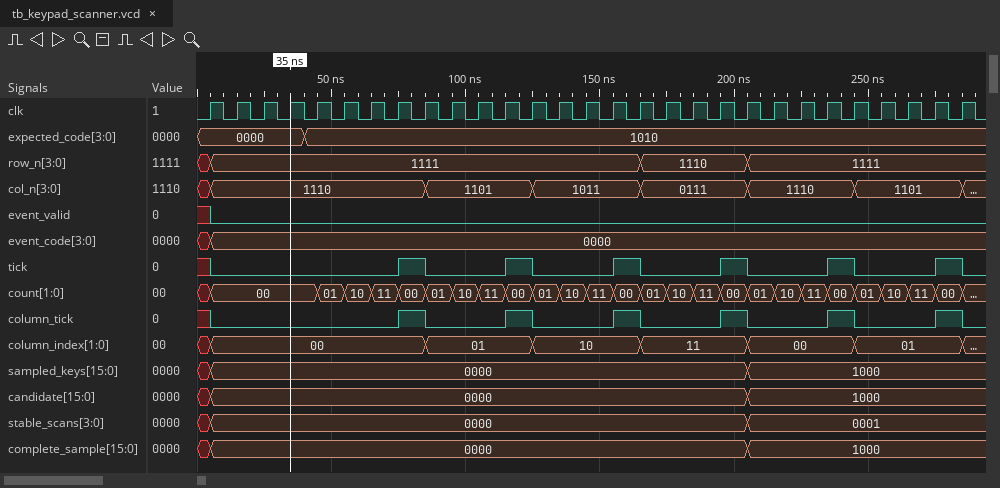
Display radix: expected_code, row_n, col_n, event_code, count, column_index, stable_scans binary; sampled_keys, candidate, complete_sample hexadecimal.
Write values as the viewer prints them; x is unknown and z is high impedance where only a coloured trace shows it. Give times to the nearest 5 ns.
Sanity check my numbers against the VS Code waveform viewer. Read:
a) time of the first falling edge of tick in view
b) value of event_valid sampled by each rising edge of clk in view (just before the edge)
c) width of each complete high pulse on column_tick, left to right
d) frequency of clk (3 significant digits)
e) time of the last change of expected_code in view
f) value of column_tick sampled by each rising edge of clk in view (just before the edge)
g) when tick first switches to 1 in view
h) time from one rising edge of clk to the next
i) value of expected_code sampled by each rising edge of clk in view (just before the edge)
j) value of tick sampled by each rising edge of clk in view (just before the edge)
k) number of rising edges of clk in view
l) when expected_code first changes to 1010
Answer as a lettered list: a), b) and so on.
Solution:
a) 85 ns
b) x 0 0 0 0 0 0 0 0 0 0 0 0 0 0 0 0 0 0 0 0 0 0 0 0 0 0 0 0
c) 10 ns, 10 ns, 10 ns, 10 ns, 10 ns, 10 ns
d) 100 MHz
e) 40 ns
f) x 0 0 0 0 0 0 0 1 0 0 0 1 0 0 0 1 0 0 0 1 0 0 0 1 0 0 0 1
g) 75 ns
h) 10 ns
i) 0000, 0000, 0000, 0000, 1010, 1010, 1010, 1010, 1010, 1010, 1010, 1010, 1010, 1010, 1010, 1010, 1010, 1010, 1010, 1010, 1010, 1010, 1010, 1010, 1010, 1010, 1010, 1010, 1010
j) x 0 0 0 0 0 0 0 1 0 0 0 1 0 0 0 1 0 0 0 1 0 0 0 1 0 0 0 1
k) 29
l) 40 ns
